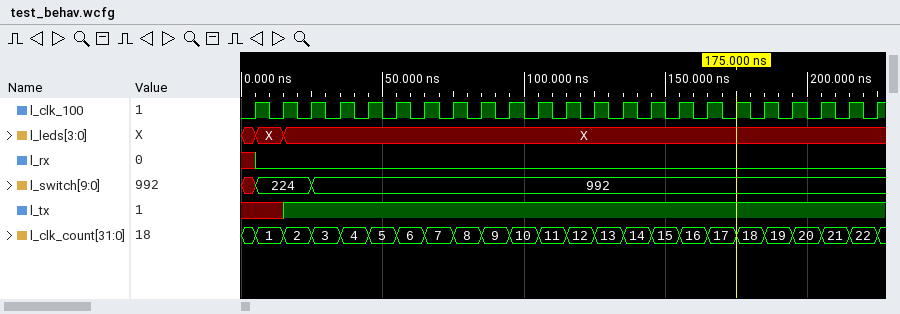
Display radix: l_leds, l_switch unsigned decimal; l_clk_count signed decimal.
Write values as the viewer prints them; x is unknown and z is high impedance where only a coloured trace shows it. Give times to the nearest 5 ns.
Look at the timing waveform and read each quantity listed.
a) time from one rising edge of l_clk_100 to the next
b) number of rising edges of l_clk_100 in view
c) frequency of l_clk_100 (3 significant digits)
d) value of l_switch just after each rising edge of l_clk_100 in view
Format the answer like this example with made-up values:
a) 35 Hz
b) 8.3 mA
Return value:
a) 10 ns
b) 23
c) 100 MHz
d) 224, 224, 992, 992, 992, 992, 992, 992, 992, 992, 992, 992, 992, 992, 992, 992, 992, 992, 992, 992, 992, 992, 992
